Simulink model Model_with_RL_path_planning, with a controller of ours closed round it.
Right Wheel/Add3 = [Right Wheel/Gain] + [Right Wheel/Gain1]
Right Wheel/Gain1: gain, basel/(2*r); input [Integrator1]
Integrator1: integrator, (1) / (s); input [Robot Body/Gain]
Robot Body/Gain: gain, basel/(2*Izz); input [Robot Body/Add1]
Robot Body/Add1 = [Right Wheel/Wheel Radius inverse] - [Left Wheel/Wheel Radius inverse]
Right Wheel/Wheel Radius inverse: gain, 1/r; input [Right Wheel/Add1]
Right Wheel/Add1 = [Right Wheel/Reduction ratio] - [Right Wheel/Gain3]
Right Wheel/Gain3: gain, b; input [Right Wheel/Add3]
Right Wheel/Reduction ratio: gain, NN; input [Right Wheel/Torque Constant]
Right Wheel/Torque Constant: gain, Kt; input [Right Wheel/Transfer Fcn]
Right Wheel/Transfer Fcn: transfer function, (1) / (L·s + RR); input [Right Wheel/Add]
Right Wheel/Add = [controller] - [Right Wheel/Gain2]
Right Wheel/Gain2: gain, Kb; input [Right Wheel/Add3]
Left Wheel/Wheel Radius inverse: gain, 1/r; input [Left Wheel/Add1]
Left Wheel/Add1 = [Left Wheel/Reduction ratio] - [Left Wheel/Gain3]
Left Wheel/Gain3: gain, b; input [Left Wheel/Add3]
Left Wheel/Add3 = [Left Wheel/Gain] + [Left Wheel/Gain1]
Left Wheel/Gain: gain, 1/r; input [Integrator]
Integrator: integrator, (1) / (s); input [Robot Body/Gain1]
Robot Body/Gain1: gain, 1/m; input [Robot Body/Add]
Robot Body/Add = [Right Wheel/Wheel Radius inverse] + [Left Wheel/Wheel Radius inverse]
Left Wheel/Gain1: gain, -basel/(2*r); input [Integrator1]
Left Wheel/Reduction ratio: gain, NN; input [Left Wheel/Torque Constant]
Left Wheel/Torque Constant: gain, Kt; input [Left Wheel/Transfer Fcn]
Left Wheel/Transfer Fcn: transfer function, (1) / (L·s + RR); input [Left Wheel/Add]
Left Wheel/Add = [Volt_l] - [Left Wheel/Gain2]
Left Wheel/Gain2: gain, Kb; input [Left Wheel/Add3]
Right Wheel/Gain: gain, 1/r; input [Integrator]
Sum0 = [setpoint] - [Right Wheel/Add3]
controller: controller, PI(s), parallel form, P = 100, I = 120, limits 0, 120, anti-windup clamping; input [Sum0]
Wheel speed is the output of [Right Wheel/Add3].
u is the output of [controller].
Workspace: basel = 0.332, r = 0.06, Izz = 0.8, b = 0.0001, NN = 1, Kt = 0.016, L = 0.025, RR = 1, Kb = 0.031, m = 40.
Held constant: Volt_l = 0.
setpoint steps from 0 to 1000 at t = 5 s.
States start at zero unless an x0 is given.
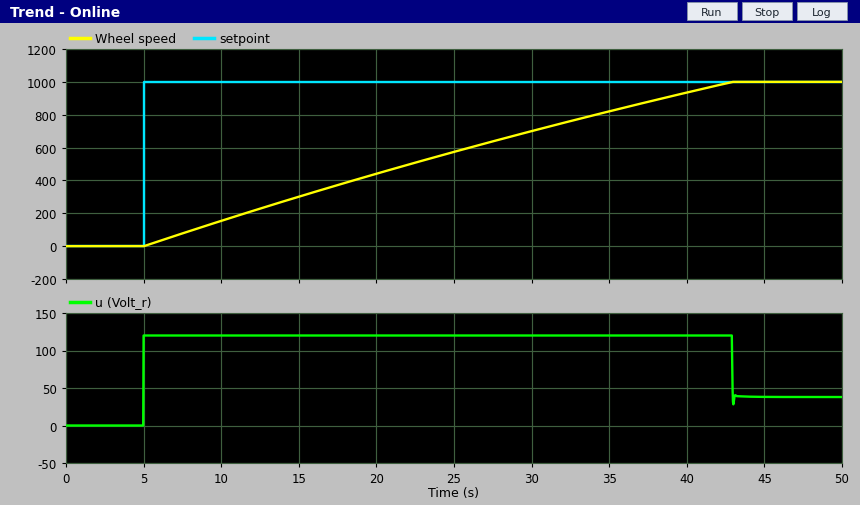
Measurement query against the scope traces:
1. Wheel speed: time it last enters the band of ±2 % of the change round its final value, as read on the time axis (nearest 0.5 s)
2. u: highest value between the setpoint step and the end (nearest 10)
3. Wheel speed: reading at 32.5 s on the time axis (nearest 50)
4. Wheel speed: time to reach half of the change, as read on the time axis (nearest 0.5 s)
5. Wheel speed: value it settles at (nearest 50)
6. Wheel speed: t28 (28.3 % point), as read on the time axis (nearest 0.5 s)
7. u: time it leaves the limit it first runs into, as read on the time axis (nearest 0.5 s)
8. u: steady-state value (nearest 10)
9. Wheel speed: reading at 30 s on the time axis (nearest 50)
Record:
42.0 s
120
750
22.0 s
1000
14.5 s
43.0 s
40
700
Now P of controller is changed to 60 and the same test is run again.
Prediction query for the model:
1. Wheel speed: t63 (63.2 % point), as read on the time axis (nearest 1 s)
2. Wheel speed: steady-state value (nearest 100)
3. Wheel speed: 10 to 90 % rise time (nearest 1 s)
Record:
27 s
1000
30 s
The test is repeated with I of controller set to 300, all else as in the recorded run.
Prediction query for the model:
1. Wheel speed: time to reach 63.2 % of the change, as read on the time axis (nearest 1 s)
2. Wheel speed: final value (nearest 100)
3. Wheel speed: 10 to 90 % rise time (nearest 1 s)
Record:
27 s
1000
30 s
